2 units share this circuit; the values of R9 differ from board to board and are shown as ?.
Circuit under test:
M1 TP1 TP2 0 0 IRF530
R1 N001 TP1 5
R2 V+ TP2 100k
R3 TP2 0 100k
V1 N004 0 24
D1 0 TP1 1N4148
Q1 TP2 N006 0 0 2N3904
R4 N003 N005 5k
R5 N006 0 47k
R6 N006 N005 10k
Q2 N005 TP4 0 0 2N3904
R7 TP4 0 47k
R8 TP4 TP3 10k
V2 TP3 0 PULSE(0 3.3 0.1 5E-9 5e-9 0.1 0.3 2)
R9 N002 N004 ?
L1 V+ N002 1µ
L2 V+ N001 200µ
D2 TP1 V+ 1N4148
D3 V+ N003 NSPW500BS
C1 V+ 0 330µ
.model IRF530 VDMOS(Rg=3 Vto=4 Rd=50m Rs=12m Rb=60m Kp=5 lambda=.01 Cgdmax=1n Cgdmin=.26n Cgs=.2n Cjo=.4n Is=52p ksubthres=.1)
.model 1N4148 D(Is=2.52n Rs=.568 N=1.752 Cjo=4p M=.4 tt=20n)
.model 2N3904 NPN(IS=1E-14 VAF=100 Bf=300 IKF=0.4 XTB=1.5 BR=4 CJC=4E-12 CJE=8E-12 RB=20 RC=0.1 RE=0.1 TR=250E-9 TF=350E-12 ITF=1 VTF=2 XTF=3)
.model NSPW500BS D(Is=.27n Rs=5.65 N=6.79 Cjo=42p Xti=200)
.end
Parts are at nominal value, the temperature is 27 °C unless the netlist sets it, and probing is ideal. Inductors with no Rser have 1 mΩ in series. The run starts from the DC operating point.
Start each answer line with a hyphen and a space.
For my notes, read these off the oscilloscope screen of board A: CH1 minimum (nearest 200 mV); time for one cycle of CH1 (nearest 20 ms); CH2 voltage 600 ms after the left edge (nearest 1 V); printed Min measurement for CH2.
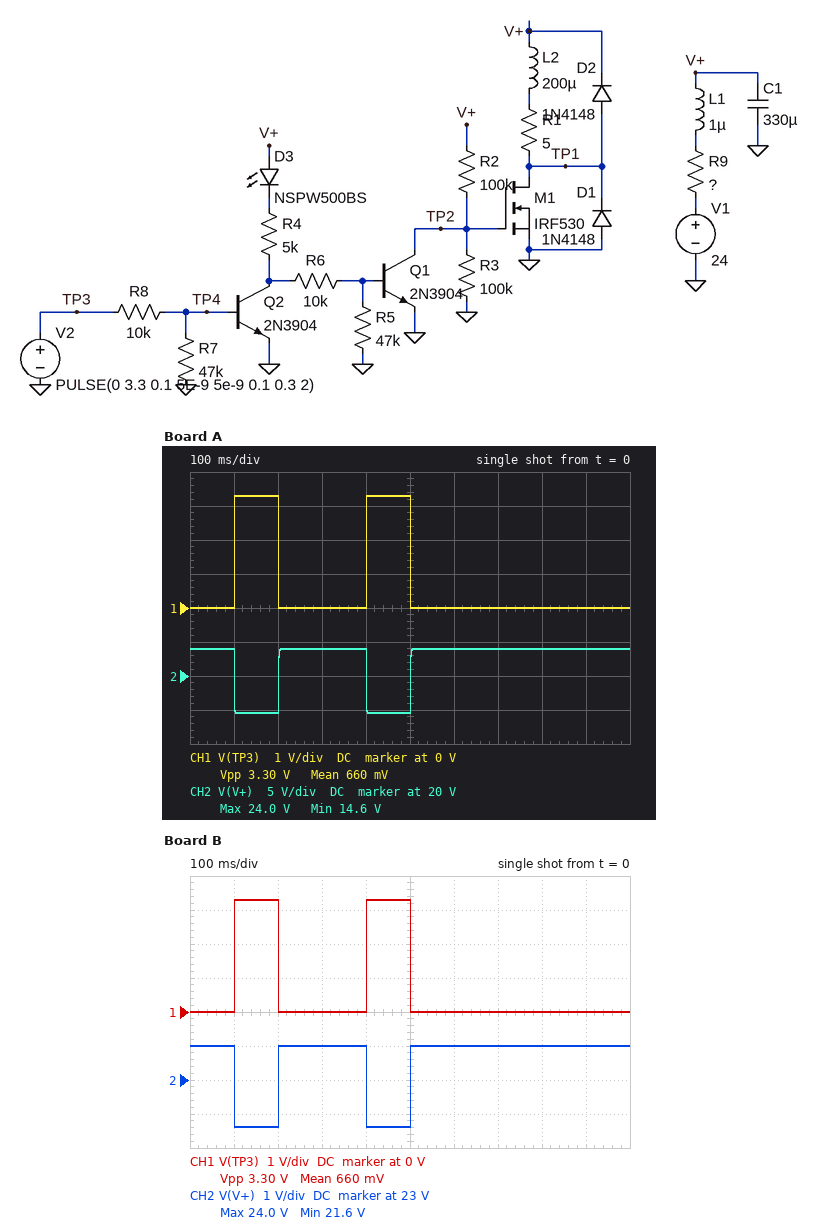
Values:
- 0 V
- 300 ms
- 24 V
- 14.6 V
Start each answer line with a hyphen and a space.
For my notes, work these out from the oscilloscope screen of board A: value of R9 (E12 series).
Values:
- 3.3 Ω
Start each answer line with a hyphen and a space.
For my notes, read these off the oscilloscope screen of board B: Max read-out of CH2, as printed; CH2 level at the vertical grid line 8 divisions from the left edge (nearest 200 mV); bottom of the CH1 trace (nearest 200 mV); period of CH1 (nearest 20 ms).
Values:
- 24.0 V
- 24.0 V
- 0 V
- 300 ms
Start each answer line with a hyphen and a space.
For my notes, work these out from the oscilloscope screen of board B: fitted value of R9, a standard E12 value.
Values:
- 0.56 Ω
